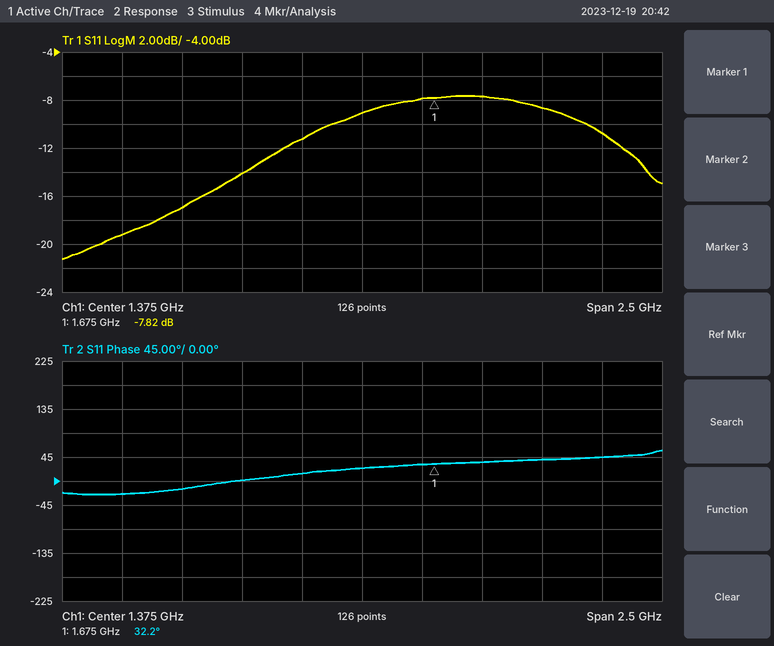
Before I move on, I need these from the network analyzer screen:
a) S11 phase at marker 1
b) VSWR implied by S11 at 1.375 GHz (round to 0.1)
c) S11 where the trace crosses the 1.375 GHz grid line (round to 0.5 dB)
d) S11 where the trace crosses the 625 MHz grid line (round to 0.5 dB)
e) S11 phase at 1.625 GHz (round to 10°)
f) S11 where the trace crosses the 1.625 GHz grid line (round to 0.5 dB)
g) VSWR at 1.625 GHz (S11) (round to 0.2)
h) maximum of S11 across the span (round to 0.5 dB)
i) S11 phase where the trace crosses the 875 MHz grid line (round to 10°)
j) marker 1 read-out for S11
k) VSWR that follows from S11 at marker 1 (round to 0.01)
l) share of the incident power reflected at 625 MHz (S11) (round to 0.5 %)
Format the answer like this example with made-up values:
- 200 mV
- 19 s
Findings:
- 32.2°
- 2.1
- -9.0 dB
- -17.0 dB
- 30°
- -8.0 dB
- 2.4
- -7.5 dB
- 0°
- -7.82 dB
- 2.37
- 2.0 %
